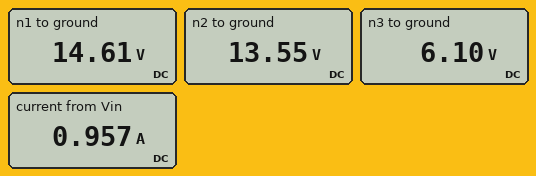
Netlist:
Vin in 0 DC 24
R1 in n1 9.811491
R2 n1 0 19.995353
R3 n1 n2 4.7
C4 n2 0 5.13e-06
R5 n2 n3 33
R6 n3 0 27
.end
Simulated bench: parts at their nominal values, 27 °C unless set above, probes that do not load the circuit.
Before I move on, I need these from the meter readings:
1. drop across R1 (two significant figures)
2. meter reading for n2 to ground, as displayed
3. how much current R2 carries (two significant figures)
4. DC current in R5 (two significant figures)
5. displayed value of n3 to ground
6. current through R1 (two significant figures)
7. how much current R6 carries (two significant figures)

9.4 V
13.55 V
730 mA
230 mA
6.10 V
960 mA
230 mA
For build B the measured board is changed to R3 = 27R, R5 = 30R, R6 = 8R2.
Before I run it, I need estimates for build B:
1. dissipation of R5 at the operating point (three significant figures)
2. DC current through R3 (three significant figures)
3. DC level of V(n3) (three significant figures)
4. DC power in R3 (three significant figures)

1.51 W
224 mA
1.84 V
1.36 W
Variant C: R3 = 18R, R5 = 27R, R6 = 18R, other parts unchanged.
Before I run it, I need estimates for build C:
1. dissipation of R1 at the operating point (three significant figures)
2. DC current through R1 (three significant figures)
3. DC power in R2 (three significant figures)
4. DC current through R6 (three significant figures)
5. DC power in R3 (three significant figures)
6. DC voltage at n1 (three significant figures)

9.05 W
960 mA
10.6 W
231 mA
964 mW
14.6 V
